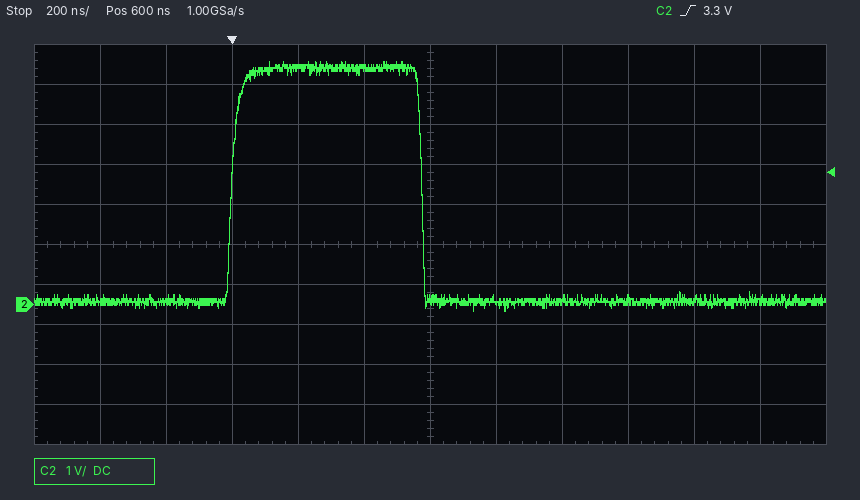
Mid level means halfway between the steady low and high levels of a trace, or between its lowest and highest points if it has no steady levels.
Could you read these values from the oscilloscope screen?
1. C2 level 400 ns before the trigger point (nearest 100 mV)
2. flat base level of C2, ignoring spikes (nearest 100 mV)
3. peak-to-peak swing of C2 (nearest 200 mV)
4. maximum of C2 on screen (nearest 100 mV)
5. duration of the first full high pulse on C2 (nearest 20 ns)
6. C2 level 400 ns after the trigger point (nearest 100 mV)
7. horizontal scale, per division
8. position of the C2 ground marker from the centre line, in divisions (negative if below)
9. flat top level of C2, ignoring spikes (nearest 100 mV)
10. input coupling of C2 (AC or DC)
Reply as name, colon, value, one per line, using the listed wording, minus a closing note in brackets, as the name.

C2 level 400 ns before the trigger point: 100 mV
flat base level of C2, ignoring spikes: 100 mV
peak-to-peak swing of C2: 6.2 V
maximum of C2 on screen: 6.1 V
duration of the first full high pulse on C2: 580 ns
C2 level 400 ns after the trigger point: 5.9 V
horizontal scale, per division: 200 ns
position of the C2 ground marker from the centre line, in divisions: -1.5 div
flat top level of C2, ignoring spikes: 5.9 V
input coupling of C2: DC
